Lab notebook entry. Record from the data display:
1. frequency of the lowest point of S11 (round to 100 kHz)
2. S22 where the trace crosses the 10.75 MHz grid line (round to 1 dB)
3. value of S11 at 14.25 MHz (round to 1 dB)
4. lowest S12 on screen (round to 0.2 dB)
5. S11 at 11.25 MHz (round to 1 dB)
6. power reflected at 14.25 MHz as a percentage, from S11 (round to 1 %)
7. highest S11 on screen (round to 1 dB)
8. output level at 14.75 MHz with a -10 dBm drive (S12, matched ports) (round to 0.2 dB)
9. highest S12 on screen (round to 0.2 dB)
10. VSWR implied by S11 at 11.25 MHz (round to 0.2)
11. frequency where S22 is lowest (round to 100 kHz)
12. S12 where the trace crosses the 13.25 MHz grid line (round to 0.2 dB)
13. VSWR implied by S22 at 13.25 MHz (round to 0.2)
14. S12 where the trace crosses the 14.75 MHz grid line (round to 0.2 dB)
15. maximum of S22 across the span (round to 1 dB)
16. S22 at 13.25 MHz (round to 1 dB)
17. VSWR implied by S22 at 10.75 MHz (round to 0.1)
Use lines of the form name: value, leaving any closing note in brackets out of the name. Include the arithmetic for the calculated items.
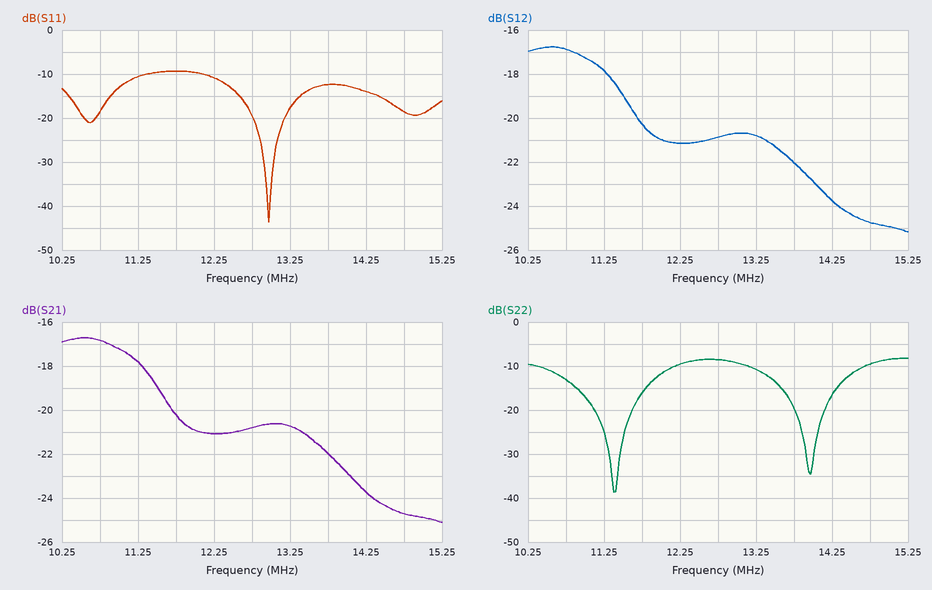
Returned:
frequency of the lowest point of S11: 13.0 MHz
S22 where the trace crosses the 10.75 MHz grid line: -13 dB
value of S11 at 14.25 MHz: -14 dB
lowest S12 on screen: -25.2 dB
S11 at 11.25 MHz: -11 dB
power reflected at 14.25 MHz as a percentage, from S11: 10^(-14/10) ≈ 4 %
highest S11 on screen: -9 dB
output level at 14.75 MHz with a -10 dBm drive (S12, matched ports): -10 dBm + (-24.8 dB) = -34.8 dBm
highest S12 on screen: -16.8 dB
VSWR implied by S11 at 11.25 MHz: |Γ| = 10^(-11/20) = 0.2818; VSWR = (1 + 0.2818)/(1 − 0.2818) ≈ 1.8
frequency where S22 is lowest: 11.4 MHz
S12 where the trace crosses the 13.25 MHz grid line: -20.8 dB
VSWR implied by S22 at 13.25 MHz: |Γ| = 10^(-11/20) = 0.2818; VSWR = (1 + 0.2818)/(1 − 0.2818) ≈ 1.8
S12 where the trace crosses the 14.75 MHz grid line: -24.8 dB
maximum of S22 across the span: -8 dB
S22 at 13.25 MHz: -11 dB
VSWR implied by S22 at 10.75 MHz: |Γ| = 10^(-13/20) = 0.2239; VSWR = (1 + 0.2239)/(1 − 0.2239) ≈ 1.6
